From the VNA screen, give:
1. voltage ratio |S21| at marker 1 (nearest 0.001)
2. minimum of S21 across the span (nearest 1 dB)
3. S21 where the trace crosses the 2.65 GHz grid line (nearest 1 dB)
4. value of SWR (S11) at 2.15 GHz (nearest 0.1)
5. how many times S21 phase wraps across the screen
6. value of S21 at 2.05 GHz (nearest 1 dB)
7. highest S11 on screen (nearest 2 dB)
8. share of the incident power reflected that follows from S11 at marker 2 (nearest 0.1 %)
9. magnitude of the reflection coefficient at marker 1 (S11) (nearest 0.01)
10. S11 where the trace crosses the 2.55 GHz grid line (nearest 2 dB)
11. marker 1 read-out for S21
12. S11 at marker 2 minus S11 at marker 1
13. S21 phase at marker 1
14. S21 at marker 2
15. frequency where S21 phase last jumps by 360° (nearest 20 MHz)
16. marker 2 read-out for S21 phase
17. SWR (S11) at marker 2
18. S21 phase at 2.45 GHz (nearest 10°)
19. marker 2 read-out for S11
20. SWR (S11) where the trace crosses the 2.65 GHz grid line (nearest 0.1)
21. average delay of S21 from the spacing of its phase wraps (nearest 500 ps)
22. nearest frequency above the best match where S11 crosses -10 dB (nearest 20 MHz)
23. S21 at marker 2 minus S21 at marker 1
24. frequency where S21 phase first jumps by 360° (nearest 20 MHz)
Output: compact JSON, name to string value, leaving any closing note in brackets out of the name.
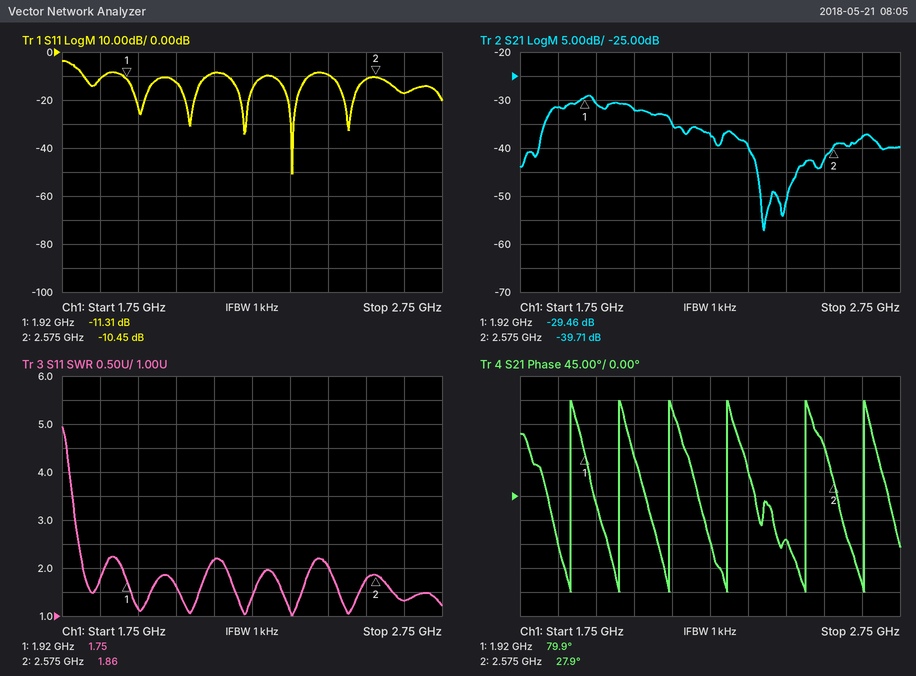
{"voltage ratio |S21| at marker 1": "0.034", "minimum of S21 across the span": "-57 dB", "S21 where the trace crosses the 2.65 GHz grid line": "-38 dB", "value of SWR (S11) at 2.15 GHz": "2.2", "how many times S21 phase wraps across the screen": "6", "value of S21 at 2.05 GHz": "-32 dB", "highest S11 on screen": "-4 dB", "share of the incident power reflected that follows from S11 at marker 2": "9.0 %", "magnitude of the reflection coefficient at marker 1 (S11)": "0.27", "S11 where the trace crosses the 2.55 GHz grid line": "-12 dB", "marker 1 read-out for S21": "-29.46 dB", "S11 at marker 2 minus S11 at marker 1": "0.86 dB", "S21 phase at marker 1": "79.9°", "S21 at marker 2": "-39.71 dB", "frequency where S21 phase last jumps by 360°": "2.66 GHz", "marker 2 read-out for S21 phase": "27.9°", "SWR (S11) at marker 2": "1.86", "S21 phase at 2.45 GHz": "-80°", "marker 2 read-out for S11": "-10.45 dB", "SWR (S11) where the trace crosses the 2.65 GHz grid line": "1.3", "average delay of S21 from the spacing of its phase wraps": "6.5 ns", "nearest frequency above the best match where S11 crosses -10 dB": "2.40 GHz", "S21 at marker 2 minus S21 at marker 1": "-10.25 dB", "frequency where S21 phase first jumps by 360°": "1.88 GHz"}
